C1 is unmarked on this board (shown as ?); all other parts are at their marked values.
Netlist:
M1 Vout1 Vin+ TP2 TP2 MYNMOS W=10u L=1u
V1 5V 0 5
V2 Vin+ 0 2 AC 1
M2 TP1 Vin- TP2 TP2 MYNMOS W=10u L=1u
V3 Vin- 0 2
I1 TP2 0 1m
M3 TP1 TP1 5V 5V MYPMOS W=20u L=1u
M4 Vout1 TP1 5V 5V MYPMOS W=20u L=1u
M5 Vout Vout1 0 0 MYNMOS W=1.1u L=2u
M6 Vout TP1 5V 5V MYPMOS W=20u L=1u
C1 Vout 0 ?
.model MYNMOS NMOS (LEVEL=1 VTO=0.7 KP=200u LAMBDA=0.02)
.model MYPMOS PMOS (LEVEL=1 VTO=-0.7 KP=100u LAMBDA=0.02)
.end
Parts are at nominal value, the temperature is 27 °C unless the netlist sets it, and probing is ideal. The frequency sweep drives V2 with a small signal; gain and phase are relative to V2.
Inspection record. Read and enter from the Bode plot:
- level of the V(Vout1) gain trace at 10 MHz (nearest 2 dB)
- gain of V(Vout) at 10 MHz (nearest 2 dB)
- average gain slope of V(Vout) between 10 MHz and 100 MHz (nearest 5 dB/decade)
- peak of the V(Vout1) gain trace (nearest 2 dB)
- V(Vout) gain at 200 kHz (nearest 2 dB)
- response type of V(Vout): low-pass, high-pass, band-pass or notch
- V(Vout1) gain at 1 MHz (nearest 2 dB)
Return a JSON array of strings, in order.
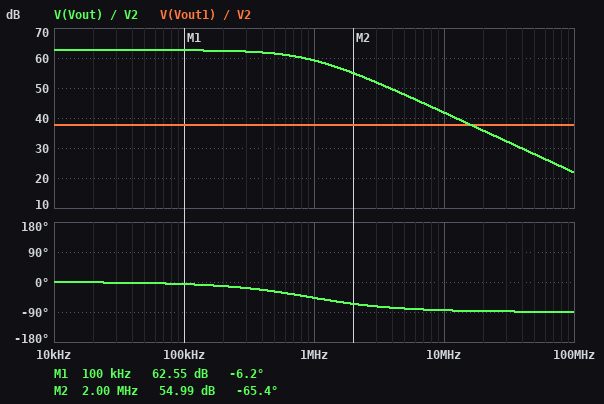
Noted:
["38 dB", "42 dB", "-20 dB/decade", "38 dB", "62 dB", "low-pass", "38 dB"]
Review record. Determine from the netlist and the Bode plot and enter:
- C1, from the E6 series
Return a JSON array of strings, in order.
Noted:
["3.3 pF"]
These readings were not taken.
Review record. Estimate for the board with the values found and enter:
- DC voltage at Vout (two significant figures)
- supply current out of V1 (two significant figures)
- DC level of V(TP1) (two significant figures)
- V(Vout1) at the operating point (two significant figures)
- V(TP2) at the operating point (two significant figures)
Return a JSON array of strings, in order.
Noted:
["3.8 V", "1.5 mA", "3.6 V", "3.6 V", "610 mV"]
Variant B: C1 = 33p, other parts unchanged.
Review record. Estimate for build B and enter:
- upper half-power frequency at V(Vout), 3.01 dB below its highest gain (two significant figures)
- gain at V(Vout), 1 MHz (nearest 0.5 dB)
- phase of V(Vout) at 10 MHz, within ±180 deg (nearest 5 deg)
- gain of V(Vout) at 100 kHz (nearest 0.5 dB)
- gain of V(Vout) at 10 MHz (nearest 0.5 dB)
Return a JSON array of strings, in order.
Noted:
["92 kHz", "42.0 dB", "-90 deg", "59.0 dB", "22.0 dB"]
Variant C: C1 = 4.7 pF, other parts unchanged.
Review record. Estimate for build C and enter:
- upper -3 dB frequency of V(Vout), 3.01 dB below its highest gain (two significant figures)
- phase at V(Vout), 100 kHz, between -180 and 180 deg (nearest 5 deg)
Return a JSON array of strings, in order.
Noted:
["640 kHz", "-10 deg"]
